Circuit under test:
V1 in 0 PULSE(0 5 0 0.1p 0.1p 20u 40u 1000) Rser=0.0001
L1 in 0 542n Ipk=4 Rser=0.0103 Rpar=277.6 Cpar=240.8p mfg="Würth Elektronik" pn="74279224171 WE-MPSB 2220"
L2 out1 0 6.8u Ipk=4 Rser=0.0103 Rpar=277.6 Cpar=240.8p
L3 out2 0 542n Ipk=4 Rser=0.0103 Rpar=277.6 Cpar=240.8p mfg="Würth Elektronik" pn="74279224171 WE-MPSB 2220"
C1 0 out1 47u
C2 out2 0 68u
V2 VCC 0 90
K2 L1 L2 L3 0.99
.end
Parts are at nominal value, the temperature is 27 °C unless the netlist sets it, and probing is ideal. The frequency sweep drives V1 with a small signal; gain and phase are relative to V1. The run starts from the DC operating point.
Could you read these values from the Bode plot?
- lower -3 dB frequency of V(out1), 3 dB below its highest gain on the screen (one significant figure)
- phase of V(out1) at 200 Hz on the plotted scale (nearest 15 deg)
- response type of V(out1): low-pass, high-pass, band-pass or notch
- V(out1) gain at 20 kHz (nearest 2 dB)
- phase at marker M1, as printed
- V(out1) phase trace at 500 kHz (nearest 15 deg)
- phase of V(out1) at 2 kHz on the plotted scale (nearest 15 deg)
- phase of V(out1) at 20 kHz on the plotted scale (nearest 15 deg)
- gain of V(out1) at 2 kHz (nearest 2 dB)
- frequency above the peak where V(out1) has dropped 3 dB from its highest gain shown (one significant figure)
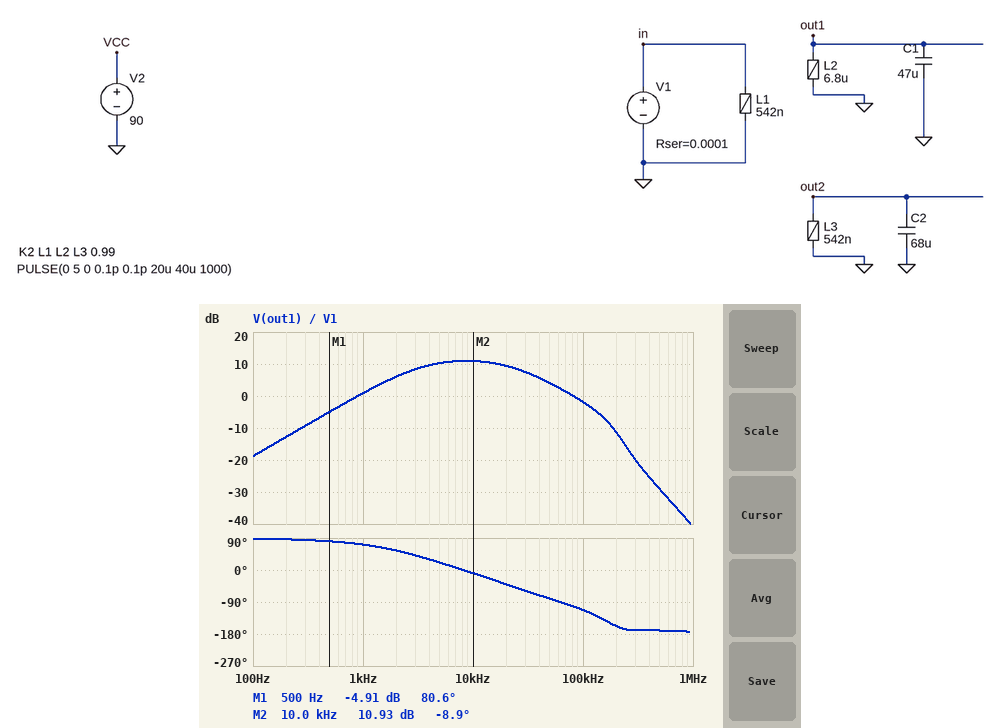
3 kHz
90 deg
band-pass
10 dB
80.6 deg
-165 deg
60 deg
-45 deg
6 dB
30 kHz
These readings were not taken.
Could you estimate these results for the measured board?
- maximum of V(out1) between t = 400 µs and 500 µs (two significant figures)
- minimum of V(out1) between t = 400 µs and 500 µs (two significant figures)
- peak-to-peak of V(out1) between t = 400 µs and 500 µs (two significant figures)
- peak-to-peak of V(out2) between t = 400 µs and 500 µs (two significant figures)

8.1 V
-8.1 V
16 V
4.5 V
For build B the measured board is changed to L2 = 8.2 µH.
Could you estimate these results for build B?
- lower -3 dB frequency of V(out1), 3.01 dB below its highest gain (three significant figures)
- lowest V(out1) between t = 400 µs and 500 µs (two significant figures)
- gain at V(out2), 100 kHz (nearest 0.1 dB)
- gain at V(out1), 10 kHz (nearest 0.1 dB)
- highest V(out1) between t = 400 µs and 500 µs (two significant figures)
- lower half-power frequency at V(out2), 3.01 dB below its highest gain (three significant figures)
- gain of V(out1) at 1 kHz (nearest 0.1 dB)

2.72 kHz
-8.4 V
-18.4 dB
11.7 dB
8.4 V
2.69 kHz
1.7 dB
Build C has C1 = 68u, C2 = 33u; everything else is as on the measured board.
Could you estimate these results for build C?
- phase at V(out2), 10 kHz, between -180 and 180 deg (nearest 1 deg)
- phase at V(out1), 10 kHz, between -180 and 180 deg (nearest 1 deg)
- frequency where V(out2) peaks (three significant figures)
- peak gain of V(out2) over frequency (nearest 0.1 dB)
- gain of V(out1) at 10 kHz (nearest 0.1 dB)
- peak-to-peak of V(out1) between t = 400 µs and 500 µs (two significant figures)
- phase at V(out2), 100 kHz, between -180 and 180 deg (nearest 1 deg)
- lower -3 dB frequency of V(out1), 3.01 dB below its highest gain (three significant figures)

-17 deg
-18 deg
7.20 kHz
-0.1 dB
10.7 dB
14 V
24 deg
2.67 kHz
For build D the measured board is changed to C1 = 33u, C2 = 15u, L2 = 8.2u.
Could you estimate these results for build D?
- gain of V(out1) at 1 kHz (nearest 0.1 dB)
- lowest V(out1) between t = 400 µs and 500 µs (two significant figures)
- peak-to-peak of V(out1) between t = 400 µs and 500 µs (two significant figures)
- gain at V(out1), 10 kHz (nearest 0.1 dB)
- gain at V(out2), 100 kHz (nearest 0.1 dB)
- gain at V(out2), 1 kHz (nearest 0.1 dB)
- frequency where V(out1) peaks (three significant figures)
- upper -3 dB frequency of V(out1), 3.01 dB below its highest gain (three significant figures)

1.7 dB
-9.4 V
19 V
11.8 dB
-24.0 dB
-10.1 dB
10.2 kHz
35.8 kHz
